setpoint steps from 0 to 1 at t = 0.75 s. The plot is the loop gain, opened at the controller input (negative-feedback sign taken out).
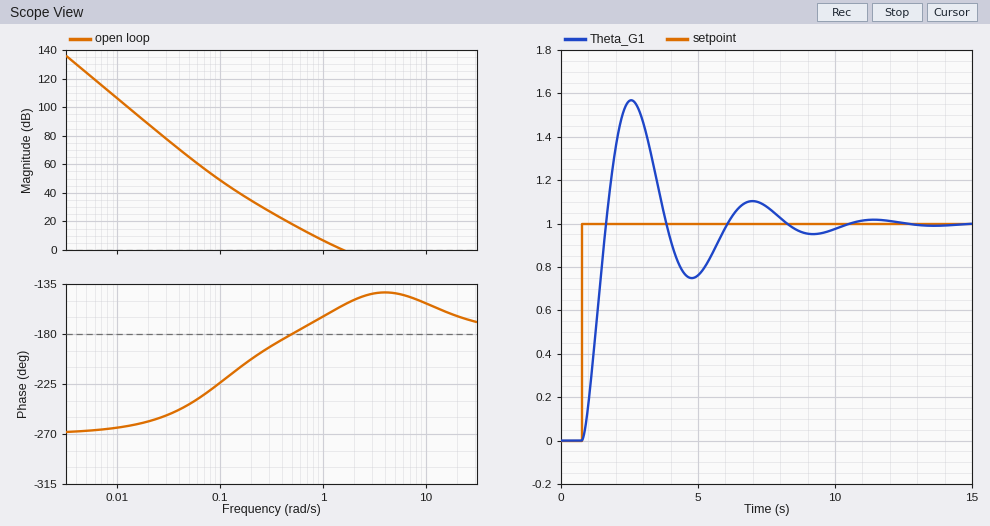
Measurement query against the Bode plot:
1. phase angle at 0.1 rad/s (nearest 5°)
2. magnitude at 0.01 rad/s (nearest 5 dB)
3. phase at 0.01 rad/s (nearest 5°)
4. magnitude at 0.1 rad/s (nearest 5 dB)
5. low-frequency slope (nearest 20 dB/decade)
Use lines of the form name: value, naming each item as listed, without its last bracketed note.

phase angle at 0.1 rad/s: -225°
magnitude at 0.01 rad/s: 105 dB
phase at 0.01 rad/s: -265°
magnitude at 0.1 rad/s: 50 dB
low-frequency slope: -60 dB/decade
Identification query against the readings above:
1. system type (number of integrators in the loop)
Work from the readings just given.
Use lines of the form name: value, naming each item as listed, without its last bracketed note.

system type: 3
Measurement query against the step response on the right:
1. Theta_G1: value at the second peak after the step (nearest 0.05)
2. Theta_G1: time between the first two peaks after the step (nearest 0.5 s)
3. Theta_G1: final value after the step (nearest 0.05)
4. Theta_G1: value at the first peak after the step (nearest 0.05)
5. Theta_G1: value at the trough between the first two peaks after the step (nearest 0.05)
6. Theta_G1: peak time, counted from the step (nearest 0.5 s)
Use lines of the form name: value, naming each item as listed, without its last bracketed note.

Theta_G1: value at the second peak after the step: 1.10
Theta_G1: time between the first two peaks after the step: 4.5 s
Theta_G1: final value after the step: 1.00
Theta_G1: value at the first peak after the step: 1.55
Theta_G1: value at the trough between the first two peaks after the step: 0.75
Theta_G1: peak time, counted from the step: 2.0 s
